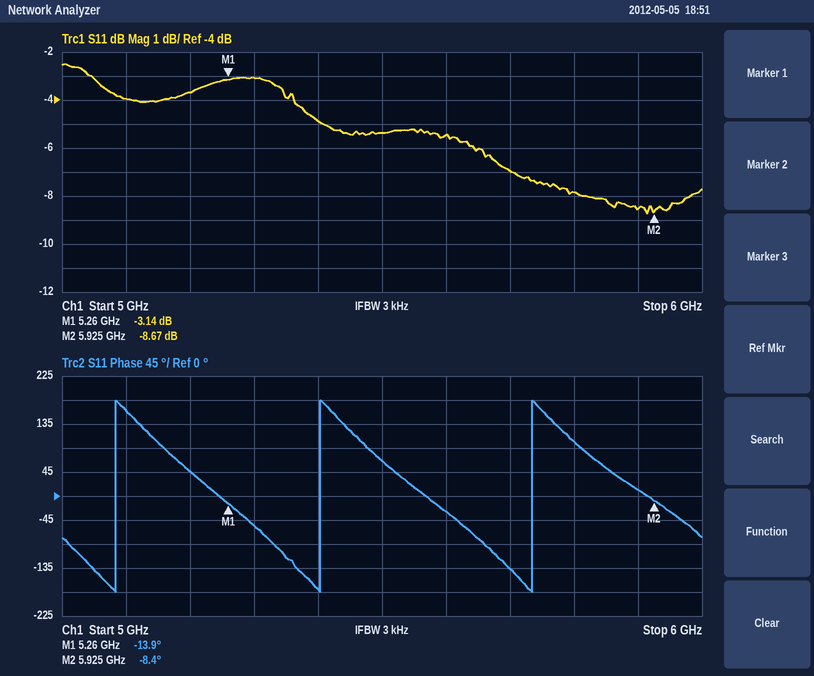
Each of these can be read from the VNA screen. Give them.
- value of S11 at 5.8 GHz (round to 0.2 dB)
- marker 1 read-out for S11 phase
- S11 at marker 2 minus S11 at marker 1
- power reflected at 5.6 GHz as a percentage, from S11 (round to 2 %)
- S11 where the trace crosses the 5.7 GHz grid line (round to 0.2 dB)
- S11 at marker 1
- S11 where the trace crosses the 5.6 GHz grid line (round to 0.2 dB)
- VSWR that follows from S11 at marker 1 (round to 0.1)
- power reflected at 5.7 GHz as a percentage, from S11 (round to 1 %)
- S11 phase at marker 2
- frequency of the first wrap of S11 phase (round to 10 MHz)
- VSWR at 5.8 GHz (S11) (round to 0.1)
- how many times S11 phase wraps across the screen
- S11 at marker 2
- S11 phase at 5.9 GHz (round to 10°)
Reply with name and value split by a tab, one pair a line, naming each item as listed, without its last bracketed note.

value of S11 at 5.8 GHz	-7.8 dB
marker 1 read-out for S11 phase	-13.9°
S11 at marker 2 minus S11 at marker 1	-5.53 dB
power reflected at 5.6 GHz as a percentage, from S11	28 %
S11 where the trace crosses the 5.7 GHz grid line	-7.0 dB
S11 at marker 1	-3.14 dB
S11 where the trace crosses the 5.6 GHz grid line	-5.4 dB
VSWR that follows from S11 at marker 1	5.6
power reflected at 5.7 GHz as a percentage, from S11	20 %
S11 phase at marker 2	-8.4°
frequency of the first wrap of S11 phase	5.08 GHz
VSWR at 5.8 GHz (S11)	2.4
how many times S11 phase wraps across the screen	3
S11 at marker 2	-8.67 dB
S11 phase at 5.9 GHz	10°
